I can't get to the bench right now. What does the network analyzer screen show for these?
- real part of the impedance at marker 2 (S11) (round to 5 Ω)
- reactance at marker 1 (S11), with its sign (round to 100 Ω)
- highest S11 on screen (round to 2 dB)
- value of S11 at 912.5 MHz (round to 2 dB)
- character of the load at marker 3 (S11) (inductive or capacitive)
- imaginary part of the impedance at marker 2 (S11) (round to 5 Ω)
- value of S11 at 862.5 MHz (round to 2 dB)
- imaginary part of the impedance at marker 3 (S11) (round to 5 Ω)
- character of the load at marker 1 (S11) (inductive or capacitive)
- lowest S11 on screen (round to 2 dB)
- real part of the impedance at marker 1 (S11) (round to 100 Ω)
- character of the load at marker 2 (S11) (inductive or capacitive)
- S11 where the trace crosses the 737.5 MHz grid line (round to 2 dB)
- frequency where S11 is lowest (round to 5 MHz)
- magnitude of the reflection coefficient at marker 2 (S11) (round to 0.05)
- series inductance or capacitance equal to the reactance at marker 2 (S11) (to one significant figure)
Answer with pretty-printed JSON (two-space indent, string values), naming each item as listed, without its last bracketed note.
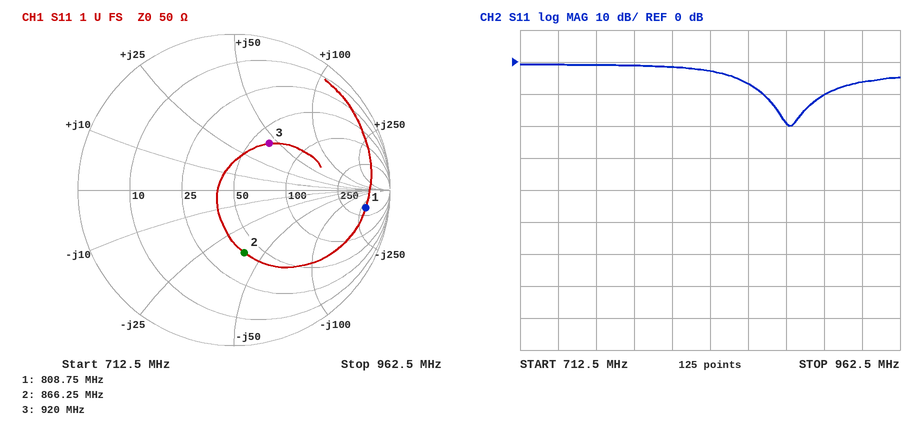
{
  "real part of the impedance at marker 2 (S11)": "40 Ω",
  "reactance at marker 1 (S11), with its sign": "-300 Ω",
  "highest S11 on screen": "0 dB",
  "value of S11 at 912.5 MHz": "-10 dB",
  "character of the load at marker 3 (S11)": "inductive",
  "imaginary part of the impedance at marker 2 (S11)": "-40 Ω",
  "value of S11 at 862.5 MHz": "-6 dB",
  "imaginary part of the impedance at marker 3 (S11)": "+45 Ω",
  "character of the load at marker 1 (S11)": "capacitive",
  "lowest S11 on screen": "-20 dB",
  "real part of the impedance at marker 1 (S11)": "400 Ω",
  "character of the load at marker 2 (S11)": "capacitive",
  "S11 where the trace crosses the 737.5 MHz grid line": "0 dB",
  "frequency where S11 is lowest": "890 MHz",
  "magnitude of the reflection coefficient at marker 2 (S11)": "0.40",
  "series inductance or capacitance equal to the reactance at marker 2 (S11)": "5 pF"
}
